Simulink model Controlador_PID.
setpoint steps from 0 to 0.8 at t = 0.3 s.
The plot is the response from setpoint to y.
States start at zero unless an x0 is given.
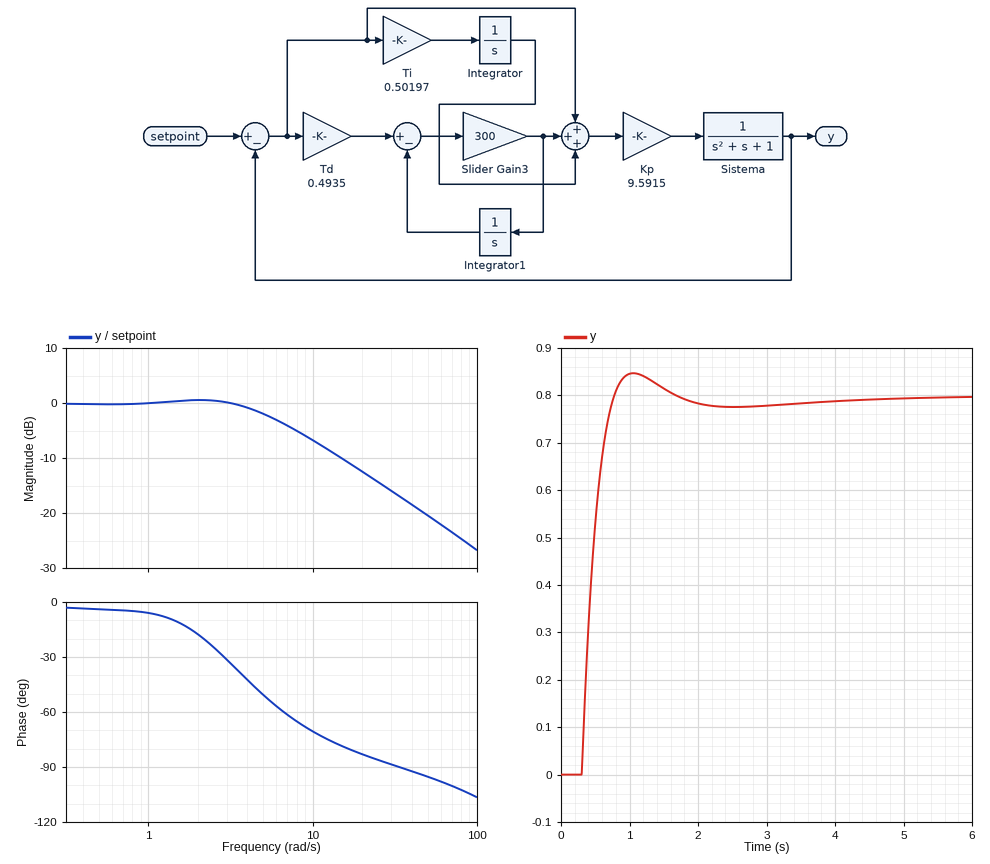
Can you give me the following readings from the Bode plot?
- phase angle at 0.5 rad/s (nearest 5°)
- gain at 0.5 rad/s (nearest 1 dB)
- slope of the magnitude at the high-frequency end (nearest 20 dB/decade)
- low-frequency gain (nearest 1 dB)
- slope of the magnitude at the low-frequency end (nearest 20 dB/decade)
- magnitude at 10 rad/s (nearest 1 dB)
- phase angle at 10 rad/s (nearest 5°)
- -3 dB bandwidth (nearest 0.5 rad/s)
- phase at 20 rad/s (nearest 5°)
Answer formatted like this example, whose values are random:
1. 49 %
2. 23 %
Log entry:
1. -5°
2. 0 dB
3. -20 dB/decade
4. 0 dB
5. 0 dB/decade
6. -7 dB
7. -70°
8. 6.0 rad/s
9. -85°
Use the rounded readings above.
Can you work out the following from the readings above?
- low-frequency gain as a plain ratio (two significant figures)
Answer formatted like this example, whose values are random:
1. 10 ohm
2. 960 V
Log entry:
1. 1.0
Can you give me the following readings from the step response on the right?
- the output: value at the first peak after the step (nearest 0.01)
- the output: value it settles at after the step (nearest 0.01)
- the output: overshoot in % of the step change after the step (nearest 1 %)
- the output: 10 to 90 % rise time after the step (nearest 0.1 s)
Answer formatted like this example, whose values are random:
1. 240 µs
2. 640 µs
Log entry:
1. 0.85
2. 0.80
3. 6 %
4. 0.3 s
